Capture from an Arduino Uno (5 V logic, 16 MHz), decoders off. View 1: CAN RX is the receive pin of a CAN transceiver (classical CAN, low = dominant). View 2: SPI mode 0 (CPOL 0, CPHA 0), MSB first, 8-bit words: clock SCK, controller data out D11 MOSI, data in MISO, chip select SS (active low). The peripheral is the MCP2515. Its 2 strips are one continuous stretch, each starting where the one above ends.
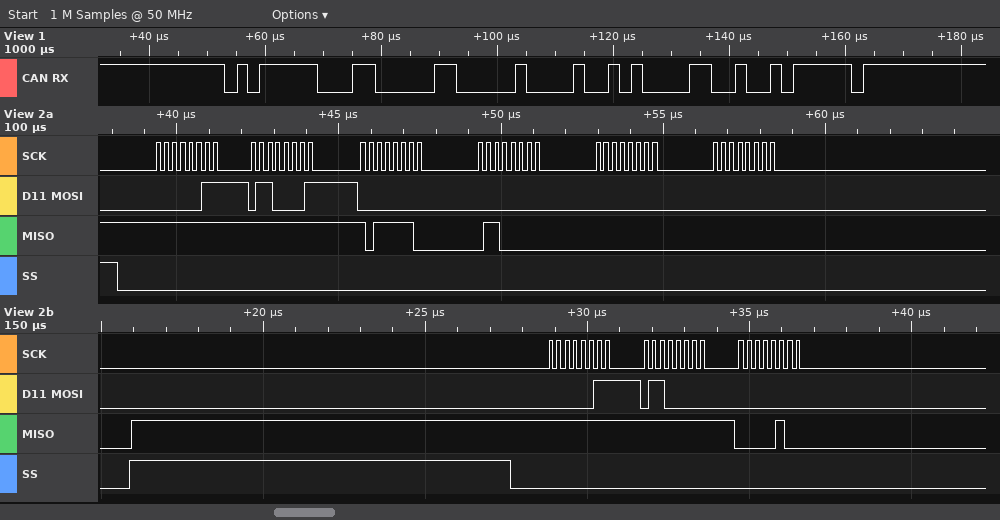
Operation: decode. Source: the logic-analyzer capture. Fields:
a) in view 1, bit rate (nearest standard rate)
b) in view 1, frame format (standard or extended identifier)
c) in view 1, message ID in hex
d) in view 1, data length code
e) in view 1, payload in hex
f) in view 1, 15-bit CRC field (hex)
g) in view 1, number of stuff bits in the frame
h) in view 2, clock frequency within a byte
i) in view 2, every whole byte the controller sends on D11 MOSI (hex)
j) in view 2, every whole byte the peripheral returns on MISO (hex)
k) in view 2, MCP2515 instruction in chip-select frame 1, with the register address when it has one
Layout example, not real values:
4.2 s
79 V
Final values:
500 kbit/s
standard
0x5F3
2
00 94
0x192F
3
4 MHz
03 61 00 00 00 00 03 60 00
FF FF BE 60 00 00 FF FF 04
READ 0x61
